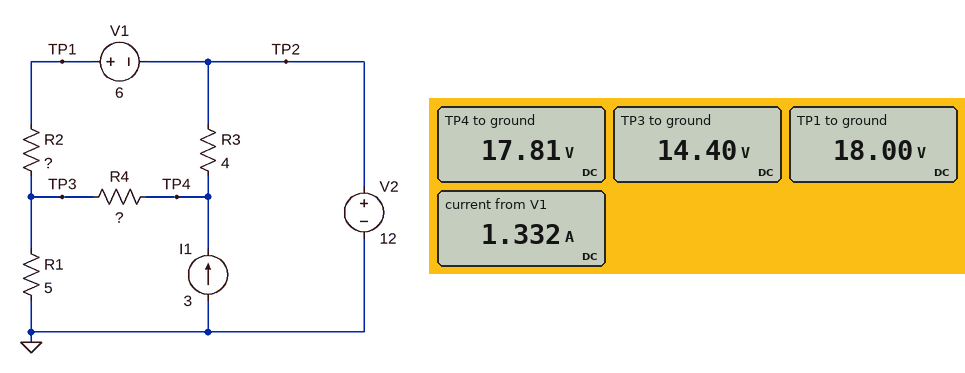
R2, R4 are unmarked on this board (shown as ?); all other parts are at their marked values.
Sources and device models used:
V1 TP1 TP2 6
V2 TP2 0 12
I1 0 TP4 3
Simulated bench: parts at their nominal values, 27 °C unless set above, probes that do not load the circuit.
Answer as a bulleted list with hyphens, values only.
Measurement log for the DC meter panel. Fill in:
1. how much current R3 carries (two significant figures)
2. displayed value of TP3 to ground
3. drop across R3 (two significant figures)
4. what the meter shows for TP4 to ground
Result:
- 1.5 A
- 14.40 V
- 5.8 V
- 17.81 V
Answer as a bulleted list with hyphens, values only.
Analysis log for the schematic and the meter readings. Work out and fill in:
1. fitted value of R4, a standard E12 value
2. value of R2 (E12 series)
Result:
- 2.2 Ω
- 2.7 Ω
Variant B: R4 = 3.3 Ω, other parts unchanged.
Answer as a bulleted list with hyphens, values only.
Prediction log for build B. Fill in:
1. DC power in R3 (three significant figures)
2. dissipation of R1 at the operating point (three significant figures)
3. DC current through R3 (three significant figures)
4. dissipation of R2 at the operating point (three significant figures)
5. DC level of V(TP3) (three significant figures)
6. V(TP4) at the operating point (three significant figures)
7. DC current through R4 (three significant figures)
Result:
- 10.8 W
- 39.6 W
- 1.64 A
- 5.71 W
- 14.1 V
- 18.6 V
- 1.36 A
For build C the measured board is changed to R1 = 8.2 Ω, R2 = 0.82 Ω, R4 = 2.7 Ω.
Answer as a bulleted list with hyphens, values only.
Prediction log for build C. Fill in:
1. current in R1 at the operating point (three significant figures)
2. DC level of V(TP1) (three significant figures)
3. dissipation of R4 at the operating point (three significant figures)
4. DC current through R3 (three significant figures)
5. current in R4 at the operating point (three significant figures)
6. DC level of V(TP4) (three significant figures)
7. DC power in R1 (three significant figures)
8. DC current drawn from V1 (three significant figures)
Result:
- 2.09 A
- 18.0 V
- 2.84 W
- 1.97 A
- 1.03 A
- 19.9 V
- 35.8 W
- 1.06 A
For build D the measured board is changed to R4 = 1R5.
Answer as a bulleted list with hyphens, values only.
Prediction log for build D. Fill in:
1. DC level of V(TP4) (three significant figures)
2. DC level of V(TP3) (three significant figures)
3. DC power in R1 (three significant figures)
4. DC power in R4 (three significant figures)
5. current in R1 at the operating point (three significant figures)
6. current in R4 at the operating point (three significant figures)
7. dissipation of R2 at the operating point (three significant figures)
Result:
- 17.2 V
- 14.7 V
- 43.0 W
- 4.32 W
- 2.93 A
- 1.70 A
- 4.12 W
